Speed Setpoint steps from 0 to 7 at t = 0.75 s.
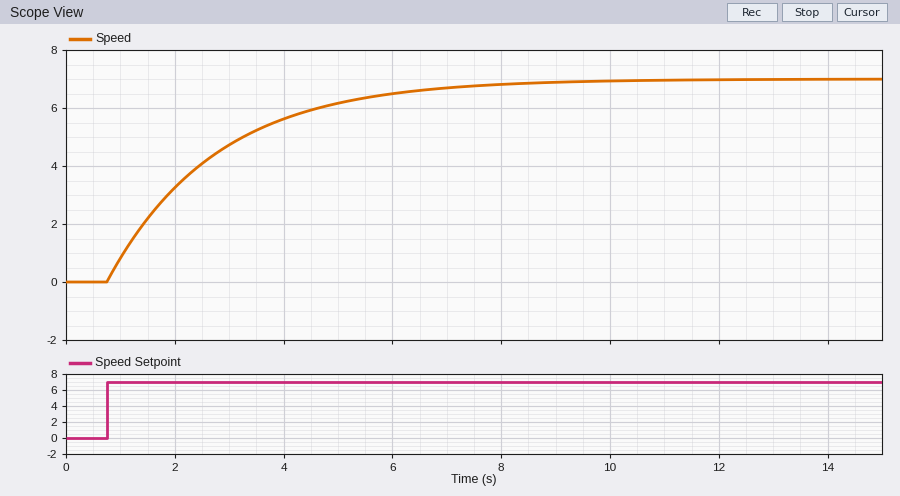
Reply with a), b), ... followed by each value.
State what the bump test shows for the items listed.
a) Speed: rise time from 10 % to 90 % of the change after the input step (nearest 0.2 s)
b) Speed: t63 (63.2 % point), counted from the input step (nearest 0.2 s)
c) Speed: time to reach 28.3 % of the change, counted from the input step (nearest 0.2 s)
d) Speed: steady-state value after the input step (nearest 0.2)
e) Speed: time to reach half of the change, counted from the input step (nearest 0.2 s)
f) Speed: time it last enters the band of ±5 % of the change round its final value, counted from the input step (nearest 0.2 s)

a) 4.4 s
b) 2.0 s
c) 0.6 s
d) 7.0
e) 1.4 s
f) 6.0 s
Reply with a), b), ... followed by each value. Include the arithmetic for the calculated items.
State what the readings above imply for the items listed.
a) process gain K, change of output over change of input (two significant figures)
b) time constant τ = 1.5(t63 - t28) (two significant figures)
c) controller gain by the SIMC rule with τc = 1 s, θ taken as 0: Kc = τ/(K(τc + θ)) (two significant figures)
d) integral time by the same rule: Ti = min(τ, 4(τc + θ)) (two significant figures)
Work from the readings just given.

a) (7 - 0) / 7 = 1.0
b) 1.5 × (2 - 0.6) = 2.1 s
c) 2.1 / (1 × (1 + 0)) = 2.1
d) min(2.1, 4 × (1 + 0)) = 2.1 s
